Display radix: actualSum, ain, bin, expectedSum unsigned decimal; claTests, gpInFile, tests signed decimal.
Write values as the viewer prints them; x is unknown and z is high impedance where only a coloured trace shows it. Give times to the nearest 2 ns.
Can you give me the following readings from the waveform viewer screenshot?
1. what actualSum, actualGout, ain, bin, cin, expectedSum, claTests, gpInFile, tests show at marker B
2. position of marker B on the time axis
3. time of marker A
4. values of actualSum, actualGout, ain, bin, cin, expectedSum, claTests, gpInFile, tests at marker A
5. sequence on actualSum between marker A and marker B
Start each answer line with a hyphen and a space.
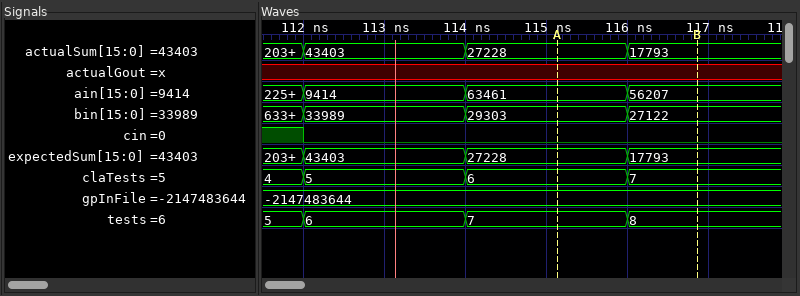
- actualSum=17793, actualGout=x, ain=56207, bin=27122, cin=0, expectedSum=17793, claTests=7, gpInFile=-2147483644, tests=8
- 116 ns
- 116 ns
- actualSum=27228, actualGout=x, ain=63461, bin=29303, cin=0, expectedSum=27228, claTests=6, gpInFile=-2147483644, tests=7
- 27228, 17793
